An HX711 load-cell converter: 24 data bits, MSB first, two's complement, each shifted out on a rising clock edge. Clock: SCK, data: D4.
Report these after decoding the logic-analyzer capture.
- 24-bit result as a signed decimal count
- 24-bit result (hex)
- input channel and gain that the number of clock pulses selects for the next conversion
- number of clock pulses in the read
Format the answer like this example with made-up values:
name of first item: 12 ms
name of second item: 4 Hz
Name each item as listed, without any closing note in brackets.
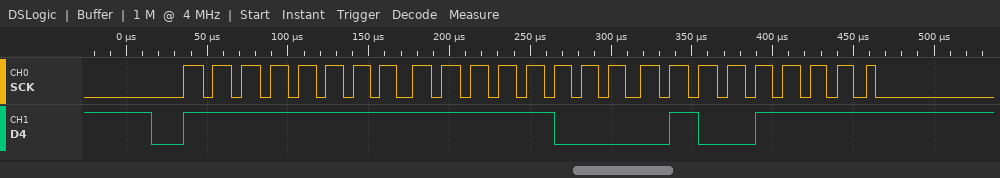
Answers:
24-bit result as a signed decimal count: -1969
24-bit result: 0xFFF84F
input channel and gain that the number of clock pulses selects for the next conversion: channel A, gain 128
number of clock pulses in the read: 25
